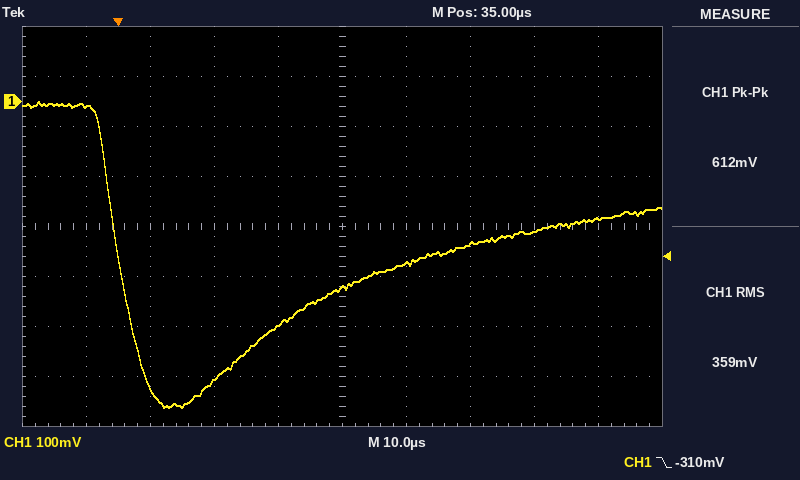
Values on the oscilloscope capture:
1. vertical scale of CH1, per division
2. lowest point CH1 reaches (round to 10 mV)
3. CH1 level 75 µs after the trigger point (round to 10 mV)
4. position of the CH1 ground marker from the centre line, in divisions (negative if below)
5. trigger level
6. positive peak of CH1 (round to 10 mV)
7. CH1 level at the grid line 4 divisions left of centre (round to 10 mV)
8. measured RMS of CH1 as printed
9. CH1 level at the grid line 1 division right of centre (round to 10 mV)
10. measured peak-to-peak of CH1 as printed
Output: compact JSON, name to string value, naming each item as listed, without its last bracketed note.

{"vertical scale of CH1, per division": "100 mV", "lowest point CH1 reaches": "-610 mV", "CH1 level 75 µs after the trigger point": "-230 mV", "position of the CH1 ground marker from the centre line, in divisions": "+2.5 div", "trigger level": "-310 mV", "positive peak of CH1": "0 mV", "CH1 level at the grid line 4 divisions left of centre": "-10 mV", "measured RMS of CH1 as printed": "359 mV", "CH1 level at the grid line 1 division right of centre": "-320 mV", "measured peak-to-peak of CH1 as printed": "612 mV"}
